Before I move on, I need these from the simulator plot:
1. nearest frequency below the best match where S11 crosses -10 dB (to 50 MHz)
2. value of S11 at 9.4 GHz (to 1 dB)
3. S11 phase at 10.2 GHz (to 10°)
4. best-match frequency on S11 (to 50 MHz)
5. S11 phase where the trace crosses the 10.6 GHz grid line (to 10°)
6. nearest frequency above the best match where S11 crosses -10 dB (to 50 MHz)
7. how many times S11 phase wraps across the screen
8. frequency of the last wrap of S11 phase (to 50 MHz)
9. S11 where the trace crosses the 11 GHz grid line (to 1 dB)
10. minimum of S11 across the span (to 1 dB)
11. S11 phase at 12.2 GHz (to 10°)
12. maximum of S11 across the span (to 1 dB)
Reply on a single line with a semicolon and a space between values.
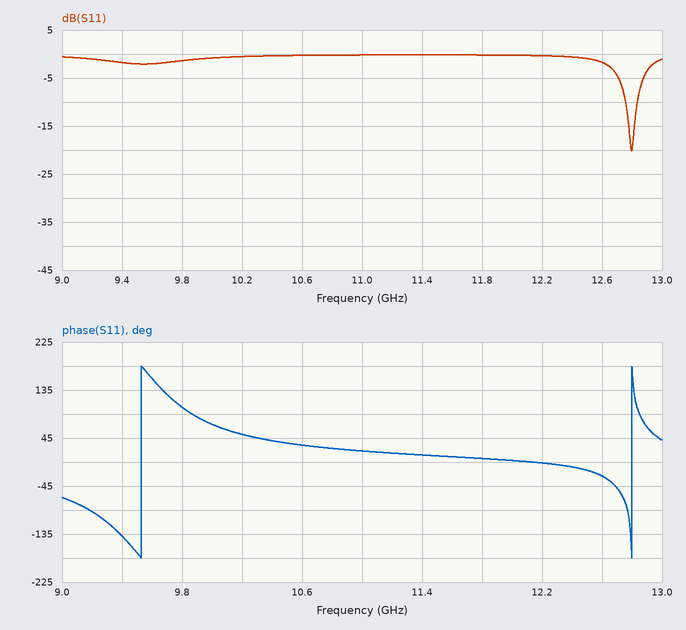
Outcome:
12.75 GHz; -2 dB; 50°; 12.80 GHz; 30°; 12.85 GHz; 2; 12.80 GHz; 0 dB; -20 dB; 0°; 0 dB
